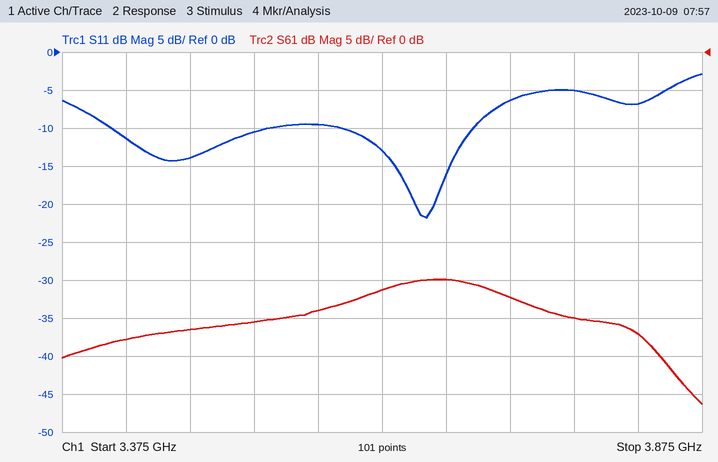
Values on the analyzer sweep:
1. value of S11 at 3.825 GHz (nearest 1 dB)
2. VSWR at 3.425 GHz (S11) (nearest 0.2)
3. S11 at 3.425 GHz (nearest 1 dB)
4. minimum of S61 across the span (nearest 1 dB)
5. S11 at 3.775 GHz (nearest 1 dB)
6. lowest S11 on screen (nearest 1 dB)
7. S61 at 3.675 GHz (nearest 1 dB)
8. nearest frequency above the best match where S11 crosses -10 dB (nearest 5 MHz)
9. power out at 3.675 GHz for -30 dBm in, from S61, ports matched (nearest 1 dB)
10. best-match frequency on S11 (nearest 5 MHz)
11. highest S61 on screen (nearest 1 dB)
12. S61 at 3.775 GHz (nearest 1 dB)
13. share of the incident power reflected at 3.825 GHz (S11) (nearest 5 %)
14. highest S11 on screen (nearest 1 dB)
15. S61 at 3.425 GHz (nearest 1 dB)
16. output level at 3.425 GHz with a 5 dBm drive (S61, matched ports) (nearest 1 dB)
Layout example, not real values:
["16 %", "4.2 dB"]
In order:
["-7 dB", "1.8", "-11 dB", "-46 dB", "-5 dB", "-22 dB", "-30 dB", "3.695 GHz", "-60 dBm", "3.660 GHz", "-30 dB", "-35 dB", "20 %", "-3 dB", "-38 dB", "-33 dBm"]
